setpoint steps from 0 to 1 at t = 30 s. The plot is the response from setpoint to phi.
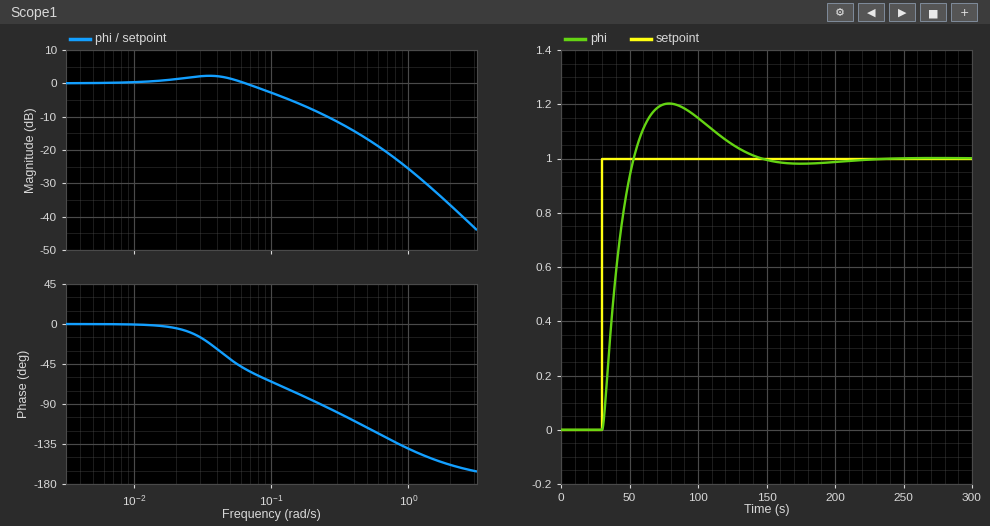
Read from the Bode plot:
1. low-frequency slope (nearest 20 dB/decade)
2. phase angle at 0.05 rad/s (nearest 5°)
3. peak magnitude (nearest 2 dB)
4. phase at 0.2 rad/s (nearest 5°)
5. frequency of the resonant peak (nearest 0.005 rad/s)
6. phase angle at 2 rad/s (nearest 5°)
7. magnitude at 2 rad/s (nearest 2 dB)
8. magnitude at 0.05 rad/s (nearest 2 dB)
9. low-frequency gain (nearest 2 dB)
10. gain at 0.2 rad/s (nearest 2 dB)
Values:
0 dB/decade
-40°
2 dB
-85°
0.035 rad/s
-160°
-36 dB
2 dB
0 dB
-8 dB
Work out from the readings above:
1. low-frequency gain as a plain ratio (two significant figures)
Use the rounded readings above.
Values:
1.0
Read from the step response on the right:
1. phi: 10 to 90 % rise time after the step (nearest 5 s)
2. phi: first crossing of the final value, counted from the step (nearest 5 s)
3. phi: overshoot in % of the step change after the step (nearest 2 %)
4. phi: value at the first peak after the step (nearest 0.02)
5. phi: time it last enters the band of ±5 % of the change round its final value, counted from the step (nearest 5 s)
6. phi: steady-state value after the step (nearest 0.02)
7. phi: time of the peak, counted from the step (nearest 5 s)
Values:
15 s
25 s
20 %
1.20
95 s
1.00
50 s
